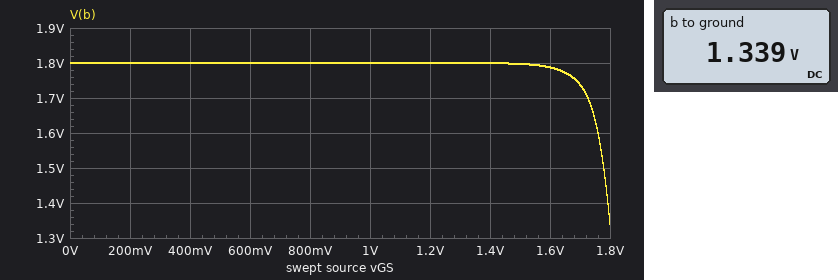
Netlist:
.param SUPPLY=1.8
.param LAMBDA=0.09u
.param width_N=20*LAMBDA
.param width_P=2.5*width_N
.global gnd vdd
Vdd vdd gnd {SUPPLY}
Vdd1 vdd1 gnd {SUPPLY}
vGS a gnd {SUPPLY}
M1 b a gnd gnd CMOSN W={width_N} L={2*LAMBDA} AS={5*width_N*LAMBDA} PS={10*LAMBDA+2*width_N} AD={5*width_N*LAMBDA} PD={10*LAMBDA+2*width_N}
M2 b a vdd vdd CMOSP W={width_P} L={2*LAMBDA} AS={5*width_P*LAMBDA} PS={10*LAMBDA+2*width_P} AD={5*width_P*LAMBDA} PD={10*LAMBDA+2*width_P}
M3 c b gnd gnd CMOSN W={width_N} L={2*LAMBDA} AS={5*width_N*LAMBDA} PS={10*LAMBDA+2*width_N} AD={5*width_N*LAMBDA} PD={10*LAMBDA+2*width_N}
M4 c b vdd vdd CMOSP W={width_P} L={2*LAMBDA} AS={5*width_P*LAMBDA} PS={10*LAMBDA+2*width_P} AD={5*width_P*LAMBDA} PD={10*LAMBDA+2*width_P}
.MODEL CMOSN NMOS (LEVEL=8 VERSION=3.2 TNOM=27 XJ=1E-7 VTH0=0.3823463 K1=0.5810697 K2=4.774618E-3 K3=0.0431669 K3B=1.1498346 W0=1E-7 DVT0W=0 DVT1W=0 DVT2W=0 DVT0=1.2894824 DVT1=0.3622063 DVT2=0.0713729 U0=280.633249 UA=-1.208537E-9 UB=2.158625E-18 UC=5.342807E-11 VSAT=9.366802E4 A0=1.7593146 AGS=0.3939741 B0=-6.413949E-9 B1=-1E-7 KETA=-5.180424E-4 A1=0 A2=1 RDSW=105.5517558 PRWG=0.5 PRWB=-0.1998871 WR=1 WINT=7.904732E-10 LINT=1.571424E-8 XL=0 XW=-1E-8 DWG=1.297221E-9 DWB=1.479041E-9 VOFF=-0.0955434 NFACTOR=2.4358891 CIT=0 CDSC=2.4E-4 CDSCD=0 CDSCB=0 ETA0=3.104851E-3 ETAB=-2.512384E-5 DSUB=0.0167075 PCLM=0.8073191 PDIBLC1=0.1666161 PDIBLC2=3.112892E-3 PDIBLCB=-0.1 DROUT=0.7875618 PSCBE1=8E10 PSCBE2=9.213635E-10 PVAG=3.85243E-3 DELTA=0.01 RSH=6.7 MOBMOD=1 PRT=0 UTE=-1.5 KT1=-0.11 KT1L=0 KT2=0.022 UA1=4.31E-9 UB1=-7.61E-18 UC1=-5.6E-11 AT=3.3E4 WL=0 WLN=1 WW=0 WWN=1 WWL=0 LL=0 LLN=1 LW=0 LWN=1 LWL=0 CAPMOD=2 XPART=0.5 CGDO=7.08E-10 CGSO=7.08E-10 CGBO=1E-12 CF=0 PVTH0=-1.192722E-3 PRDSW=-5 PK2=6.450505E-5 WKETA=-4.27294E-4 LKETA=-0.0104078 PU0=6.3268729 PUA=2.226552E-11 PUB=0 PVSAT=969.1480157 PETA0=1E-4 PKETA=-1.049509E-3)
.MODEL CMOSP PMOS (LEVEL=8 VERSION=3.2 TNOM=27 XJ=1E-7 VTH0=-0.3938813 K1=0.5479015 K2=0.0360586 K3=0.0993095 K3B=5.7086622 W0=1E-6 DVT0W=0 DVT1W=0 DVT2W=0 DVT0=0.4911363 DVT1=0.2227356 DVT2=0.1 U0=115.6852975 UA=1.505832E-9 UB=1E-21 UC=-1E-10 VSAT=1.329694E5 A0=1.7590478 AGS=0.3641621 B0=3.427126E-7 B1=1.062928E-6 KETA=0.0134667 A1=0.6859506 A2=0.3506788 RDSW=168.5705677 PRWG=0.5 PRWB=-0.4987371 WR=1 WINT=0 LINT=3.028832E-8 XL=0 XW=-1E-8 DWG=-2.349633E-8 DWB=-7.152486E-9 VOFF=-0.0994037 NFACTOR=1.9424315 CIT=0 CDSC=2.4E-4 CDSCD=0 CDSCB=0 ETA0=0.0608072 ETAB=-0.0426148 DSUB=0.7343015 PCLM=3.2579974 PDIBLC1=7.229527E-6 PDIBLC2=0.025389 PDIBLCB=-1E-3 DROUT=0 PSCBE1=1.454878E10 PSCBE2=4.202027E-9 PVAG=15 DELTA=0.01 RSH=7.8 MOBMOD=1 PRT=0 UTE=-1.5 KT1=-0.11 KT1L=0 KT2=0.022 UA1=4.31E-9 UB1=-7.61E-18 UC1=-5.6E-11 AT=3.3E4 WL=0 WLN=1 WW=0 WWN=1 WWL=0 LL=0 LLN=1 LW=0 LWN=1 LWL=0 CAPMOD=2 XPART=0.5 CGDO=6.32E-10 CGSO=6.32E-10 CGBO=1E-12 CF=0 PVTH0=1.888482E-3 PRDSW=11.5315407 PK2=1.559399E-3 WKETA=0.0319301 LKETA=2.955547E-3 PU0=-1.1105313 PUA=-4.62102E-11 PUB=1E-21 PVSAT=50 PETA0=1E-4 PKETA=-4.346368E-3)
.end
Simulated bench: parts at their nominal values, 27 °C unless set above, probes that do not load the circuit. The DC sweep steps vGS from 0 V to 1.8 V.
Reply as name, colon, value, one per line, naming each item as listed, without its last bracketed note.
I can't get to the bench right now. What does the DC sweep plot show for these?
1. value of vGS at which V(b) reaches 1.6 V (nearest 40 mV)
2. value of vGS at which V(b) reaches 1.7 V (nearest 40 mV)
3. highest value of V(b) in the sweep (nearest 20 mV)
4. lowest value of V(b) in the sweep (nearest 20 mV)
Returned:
value of vGS at which V(b) reaches 1.6 V: 1.76 V
value of vGS at which V(b) reaches 1.7 V: 1.72 V
highest value of V(b) in the sweep: 1.80 V
lowest value of V(b) in the sweep: 1.34 V
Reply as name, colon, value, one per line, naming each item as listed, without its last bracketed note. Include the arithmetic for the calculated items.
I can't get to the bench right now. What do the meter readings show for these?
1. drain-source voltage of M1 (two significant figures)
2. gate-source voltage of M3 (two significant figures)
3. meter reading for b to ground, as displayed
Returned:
drain-source voltage of M1: 1.339 V = 1.3 V
gate-source voltage of M3: 1.339 V = 1.3 V
meter reading for b to ground, as displayed: 1.339 V
